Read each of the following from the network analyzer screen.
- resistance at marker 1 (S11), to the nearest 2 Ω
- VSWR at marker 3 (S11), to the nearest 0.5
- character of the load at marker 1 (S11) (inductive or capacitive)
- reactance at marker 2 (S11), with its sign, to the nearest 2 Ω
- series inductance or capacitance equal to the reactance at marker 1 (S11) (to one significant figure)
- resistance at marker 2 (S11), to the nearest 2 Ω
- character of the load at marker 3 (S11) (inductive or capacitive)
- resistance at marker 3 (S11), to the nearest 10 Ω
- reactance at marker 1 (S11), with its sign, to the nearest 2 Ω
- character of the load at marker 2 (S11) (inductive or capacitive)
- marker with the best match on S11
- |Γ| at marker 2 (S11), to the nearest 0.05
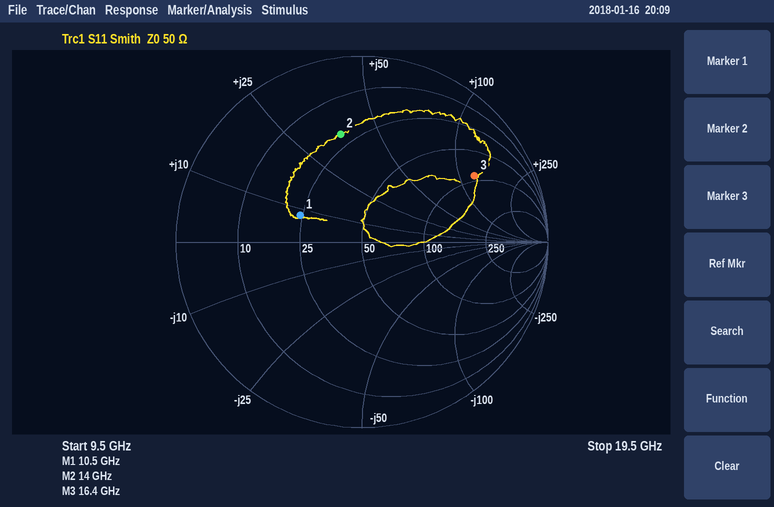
24 Ω
5.5
inductive
+36 Ω
100 pH
20 Ω
inductive
90 Ω
+8 Ω
inductive
marker 1
0.60
